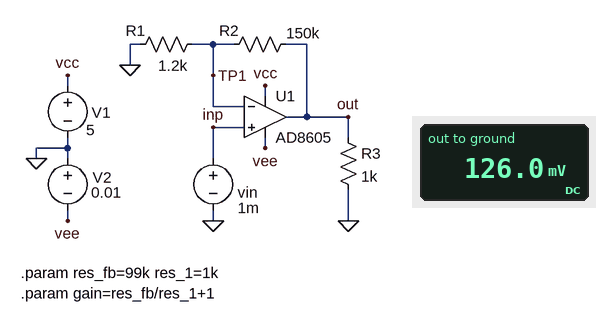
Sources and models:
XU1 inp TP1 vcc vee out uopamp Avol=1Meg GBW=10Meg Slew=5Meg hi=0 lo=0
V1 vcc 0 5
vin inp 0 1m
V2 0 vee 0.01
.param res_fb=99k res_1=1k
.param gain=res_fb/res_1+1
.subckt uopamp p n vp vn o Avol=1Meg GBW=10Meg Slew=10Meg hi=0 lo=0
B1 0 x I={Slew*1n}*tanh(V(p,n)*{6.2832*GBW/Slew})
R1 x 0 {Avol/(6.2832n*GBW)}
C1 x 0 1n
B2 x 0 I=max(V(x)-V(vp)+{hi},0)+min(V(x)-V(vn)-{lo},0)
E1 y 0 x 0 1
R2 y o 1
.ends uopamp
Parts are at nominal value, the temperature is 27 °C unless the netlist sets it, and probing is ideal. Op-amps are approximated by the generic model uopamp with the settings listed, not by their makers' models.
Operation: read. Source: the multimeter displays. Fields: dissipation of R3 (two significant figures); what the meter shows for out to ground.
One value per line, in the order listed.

16 µW
126.0 mV
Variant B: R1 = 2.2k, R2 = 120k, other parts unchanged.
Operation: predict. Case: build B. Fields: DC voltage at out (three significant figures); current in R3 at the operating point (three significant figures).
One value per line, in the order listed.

55.5 mV
55.5 µA
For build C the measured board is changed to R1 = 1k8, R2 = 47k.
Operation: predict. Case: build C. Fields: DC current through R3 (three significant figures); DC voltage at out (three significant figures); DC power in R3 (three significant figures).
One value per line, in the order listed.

27.1 µA
27.1 mV
735 nW
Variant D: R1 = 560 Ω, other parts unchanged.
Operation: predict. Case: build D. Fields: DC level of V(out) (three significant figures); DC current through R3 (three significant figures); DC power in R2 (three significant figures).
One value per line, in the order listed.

269 mV
269 µA
478 nW
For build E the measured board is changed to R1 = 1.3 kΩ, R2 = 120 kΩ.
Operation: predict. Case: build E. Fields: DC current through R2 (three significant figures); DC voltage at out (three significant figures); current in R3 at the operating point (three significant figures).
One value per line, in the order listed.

769 nA
93.3 mV
93.3 µA
